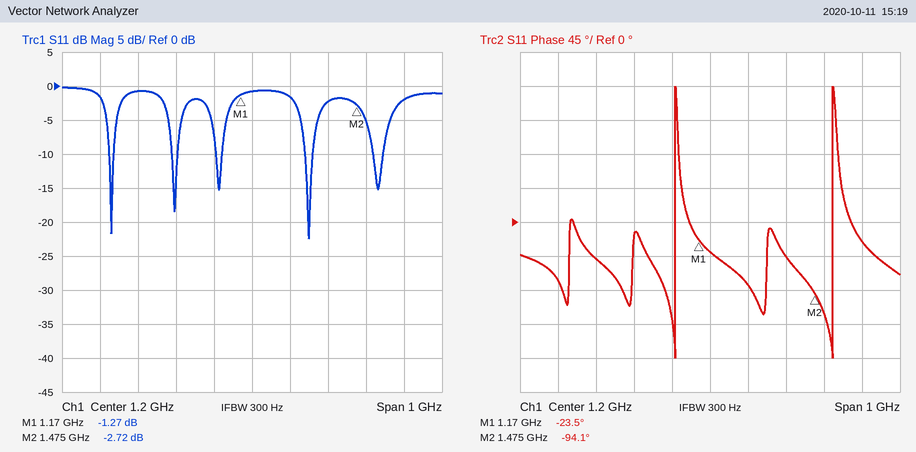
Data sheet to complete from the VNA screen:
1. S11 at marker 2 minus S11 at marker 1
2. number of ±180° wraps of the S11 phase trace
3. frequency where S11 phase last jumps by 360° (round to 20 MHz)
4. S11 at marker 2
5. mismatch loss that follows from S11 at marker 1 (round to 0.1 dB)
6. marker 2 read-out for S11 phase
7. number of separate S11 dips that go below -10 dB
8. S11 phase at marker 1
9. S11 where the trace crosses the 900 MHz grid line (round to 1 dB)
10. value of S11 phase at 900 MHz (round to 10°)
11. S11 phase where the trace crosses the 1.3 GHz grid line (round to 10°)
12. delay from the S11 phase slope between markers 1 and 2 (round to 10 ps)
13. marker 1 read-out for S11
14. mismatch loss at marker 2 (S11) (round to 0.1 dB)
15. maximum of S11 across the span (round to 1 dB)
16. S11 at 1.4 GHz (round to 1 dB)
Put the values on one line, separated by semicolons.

-1.45 dB; 2; 1.52 GHz; -2.72 dB; 6.0 dB; -94.1°; 5; -23.5°; -1 dB; -50°; -80°; 640 ps; -1.27 dB; 3.3 dB; 0 dB; -2 dB
